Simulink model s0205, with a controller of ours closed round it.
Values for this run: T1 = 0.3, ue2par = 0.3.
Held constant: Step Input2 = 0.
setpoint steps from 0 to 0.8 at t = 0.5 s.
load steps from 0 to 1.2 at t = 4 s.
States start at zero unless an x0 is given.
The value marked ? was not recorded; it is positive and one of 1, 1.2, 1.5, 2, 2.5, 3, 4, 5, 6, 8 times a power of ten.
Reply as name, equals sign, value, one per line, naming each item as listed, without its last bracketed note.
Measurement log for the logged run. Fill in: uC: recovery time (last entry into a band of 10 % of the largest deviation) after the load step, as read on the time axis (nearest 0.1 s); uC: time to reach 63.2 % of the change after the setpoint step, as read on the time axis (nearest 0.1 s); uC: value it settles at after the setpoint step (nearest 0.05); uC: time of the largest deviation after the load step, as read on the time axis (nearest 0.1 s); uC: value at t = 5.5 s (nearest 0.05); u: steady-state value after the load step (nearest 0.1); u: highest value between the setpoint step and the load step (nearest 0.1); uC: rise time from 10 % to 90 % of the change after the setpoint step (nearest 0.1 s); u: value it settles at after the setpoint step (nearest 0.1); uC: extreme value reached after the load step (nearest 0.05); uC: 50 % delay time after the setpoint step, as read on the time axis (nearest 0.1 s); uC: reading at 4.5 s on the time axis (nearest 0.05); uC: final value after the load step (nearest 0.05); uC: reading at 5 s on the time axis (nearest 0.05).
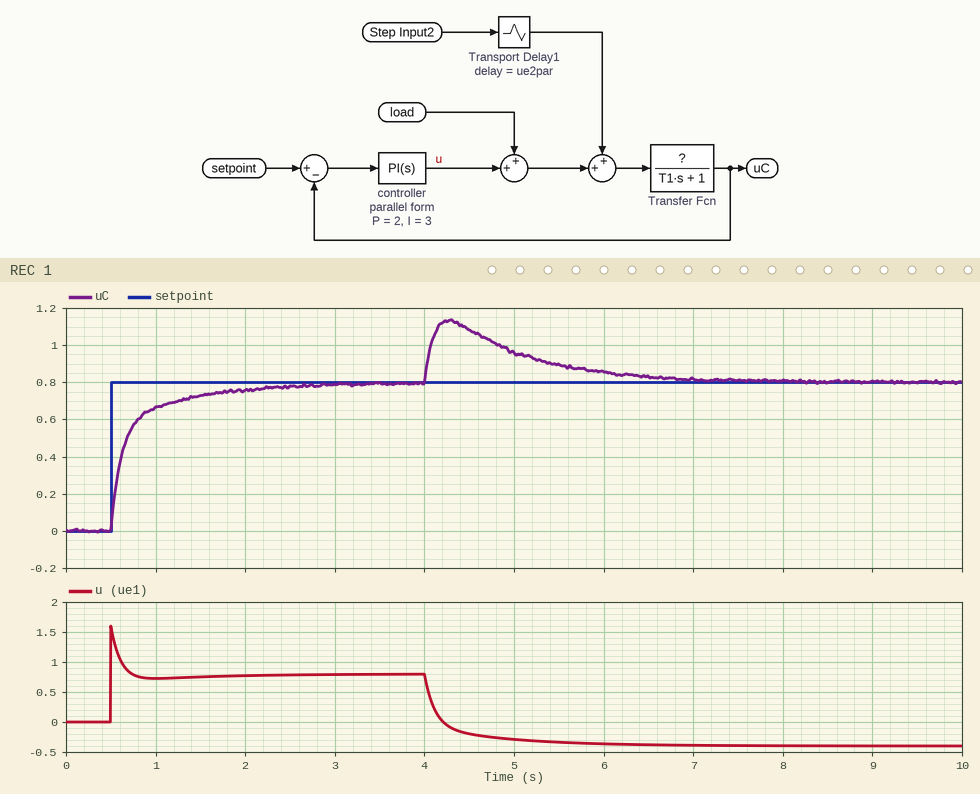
uC: recovery time (last entry into a band of 10 % of the largest deviation) after the load step, as read on the time axis = 6.4 s
uC: time to reach 63.2 % of the change after the setpoint step, as read on the time axis = 0.7 s
uC: value it settles at after the setpoint step = 0.80
uC: time of the largest deviation after the load step, as read on the time axis = 4.3 s
uC: value at t = 5.5 s = 0.90
u: steady-state value after the load step = -0.4
u: highest value between the setpoint step and the load step = 1.6
uC: rise time from 10 % to 90 % of the change after the setpoint step = 0.9 s
u: value it settles at after the setpoint step = 0.8
uC: extreme value reached after the load step = 1.15
uC: 50 % delay time after the setpoint step, as read on the time axis = 0.6 s
uC: reading at 4.5 s on the time axis = 1.10
uC: final value after the load step = 0.80
uC: reading at 5 s on the time axis = 0.95
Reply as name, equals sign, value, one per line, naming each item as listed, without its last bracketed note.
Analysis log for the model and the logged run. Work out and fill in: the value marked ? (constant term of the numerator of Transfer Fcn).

the value marked ? = 1
